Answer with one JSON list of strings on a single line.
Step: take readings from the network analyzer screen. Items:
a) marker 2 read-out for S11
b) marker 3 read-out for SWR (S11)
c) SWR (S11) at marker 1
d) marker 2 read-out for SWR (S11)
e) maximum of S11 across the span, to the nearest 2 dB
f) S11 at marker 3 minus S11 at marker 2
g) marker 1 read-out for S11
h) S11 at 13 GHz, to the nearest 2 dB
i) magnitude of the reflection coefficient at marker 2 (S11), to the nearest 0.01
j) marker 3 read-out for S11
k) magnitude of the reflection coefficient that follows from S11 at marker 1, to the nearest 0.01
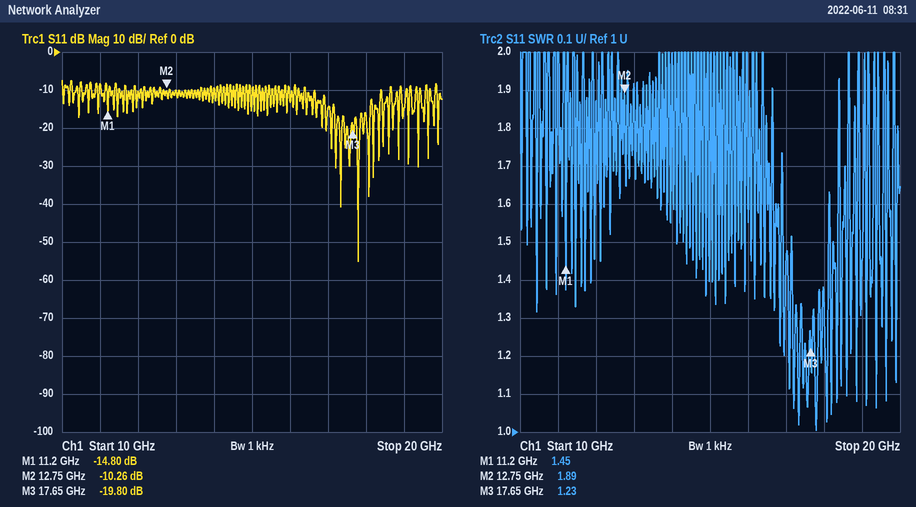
["-10.26 dB", "1.23", "1.45", "1.89", "-8 dB", "-9.54 dB", "-14.80 dB", "-10 dB", "0.31", "-19.80 dB", "0.18"]
